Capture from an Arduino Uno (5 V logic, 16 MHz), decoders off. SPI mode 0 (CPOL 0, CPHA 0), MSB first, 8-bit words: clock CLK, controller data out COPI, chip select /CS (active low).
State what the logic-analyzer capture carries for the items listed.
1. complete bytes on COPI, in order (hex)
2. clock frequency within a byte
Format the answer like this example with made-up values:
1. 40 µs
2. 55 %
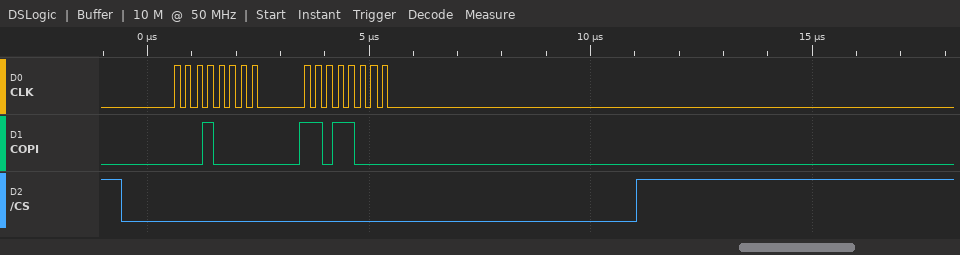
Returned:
1. 0x10 0xD8
2. 4 MHz
